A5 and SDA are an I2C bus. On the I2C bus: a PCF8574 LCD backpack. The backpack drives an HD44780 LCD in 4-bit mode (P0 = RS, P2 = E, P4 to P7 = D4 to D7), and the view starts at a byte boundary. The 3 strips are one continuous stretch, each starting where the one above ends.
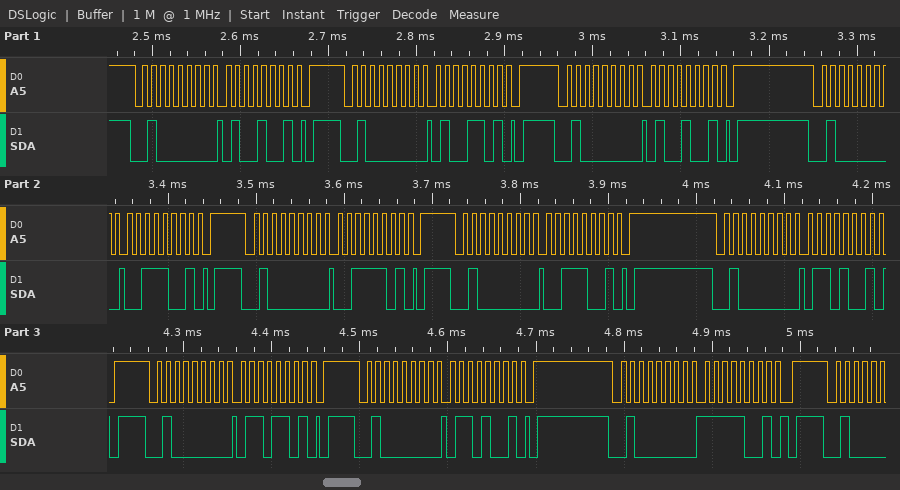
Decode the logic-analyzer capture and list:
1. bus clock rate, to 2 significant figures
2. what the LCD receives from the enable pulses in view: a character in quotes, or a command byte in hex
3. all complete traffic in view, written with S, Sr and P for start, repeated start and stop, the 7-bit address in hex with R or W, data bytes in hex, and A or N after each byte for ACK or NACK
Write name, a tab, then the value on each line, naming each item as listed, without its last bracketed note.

bus clock rate, to 2 significant figures	100 kHz
what the LCD receives from the enable pulses in view: a character in quotes, or a command byte in hex	'C'
all complete traffic in view, written with S, Sr and P for start, repeated start and stop, the 7-bit address in hex with R or W, data bytes in hex, and A or N after each byte for ACK or NACK	S 20W A 49 A P S 20W A 4D A P S 20W A 49 A P S 20W A 39 A P S 20W A 3D A P S 20W A 39 A P S 20W A 69 A P S 20W A 6D A P S 20W A 69 A P S 20W A F9 A P
